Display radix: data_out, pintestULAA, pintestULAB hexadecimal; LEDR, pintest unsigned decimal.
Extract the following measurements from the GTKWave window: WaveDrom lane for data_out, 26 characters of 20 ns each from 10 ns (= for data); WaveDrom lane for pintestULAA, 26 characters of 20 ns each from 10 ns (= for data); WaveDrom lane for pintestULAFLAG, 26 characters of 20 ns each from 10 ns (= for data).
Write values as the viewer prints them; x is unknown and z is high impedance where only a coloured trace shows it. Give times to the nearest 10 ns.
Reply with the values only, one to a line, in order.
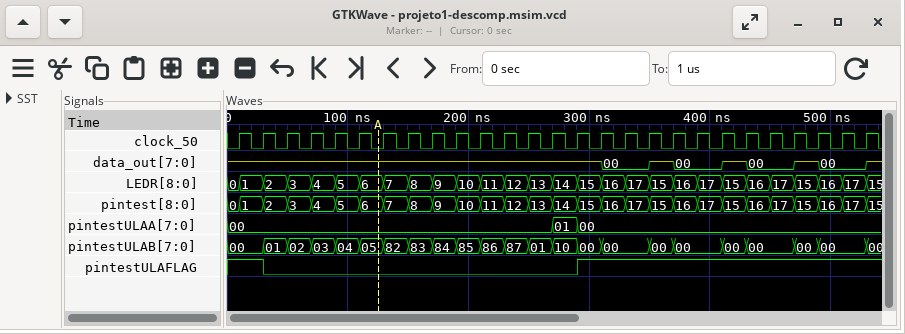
{name: 'data_out', wave: 'z..............=.z=.z=.z=.', data: '00 00 00 00'}
{name: 'pintestULAA', wave: '=............==...........', data: '00 01 00'}
{name: 'pintestULAFLAG', wave: '10............1...........'}
